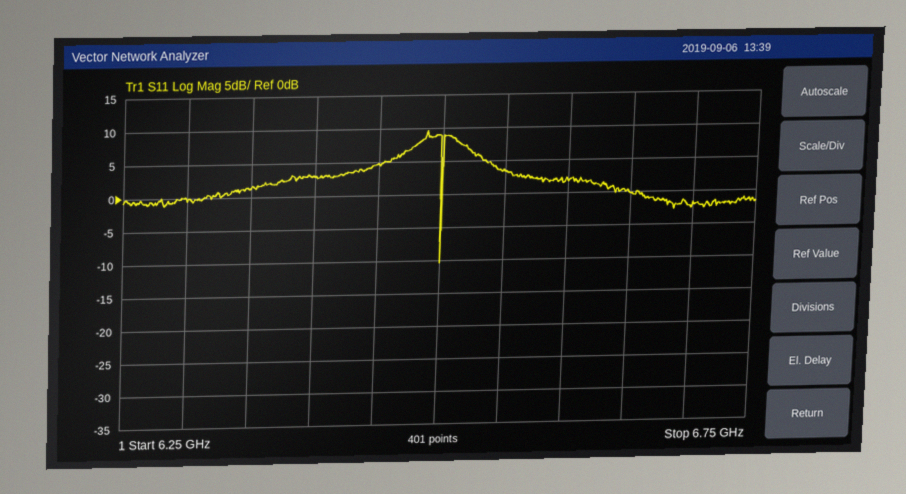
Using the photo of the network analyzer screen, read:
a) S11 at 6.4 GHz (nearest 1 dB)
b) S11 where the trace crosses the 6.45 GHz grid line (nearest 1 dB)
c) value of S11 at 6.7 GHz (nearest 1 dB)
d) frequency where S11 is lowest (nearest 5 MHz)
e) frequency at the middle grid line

3 dB
5 dB
-2 dB
6.500 GHz
6.5 GHz
